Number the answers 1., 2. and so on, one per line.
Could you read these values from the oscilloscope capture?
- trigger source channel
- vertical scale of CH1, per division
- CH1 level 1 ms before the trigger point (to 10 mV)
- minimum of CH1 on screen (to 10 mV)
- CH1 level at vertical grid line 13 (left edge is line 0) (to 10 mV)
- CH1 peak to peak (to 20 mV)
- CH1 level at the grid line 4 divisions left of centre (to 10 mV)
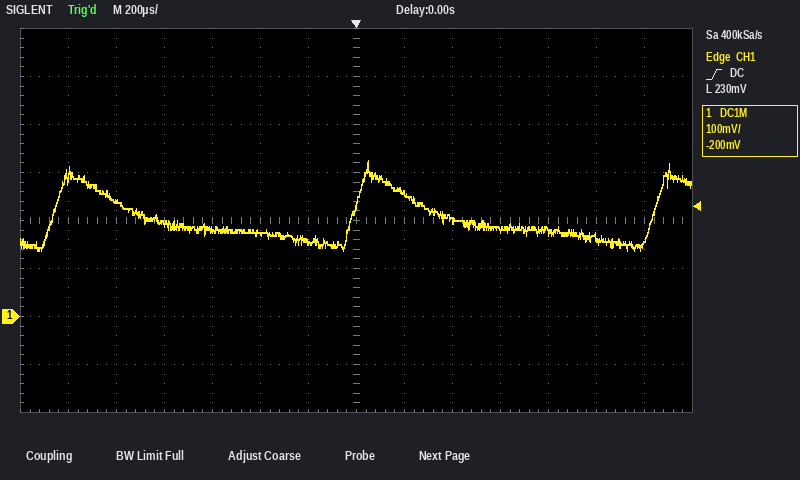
1. CH1
2. 100 mV
3. 240 mV
4. 140 mV
5. 150 mV
6. 180 mV
7. 190 mV
